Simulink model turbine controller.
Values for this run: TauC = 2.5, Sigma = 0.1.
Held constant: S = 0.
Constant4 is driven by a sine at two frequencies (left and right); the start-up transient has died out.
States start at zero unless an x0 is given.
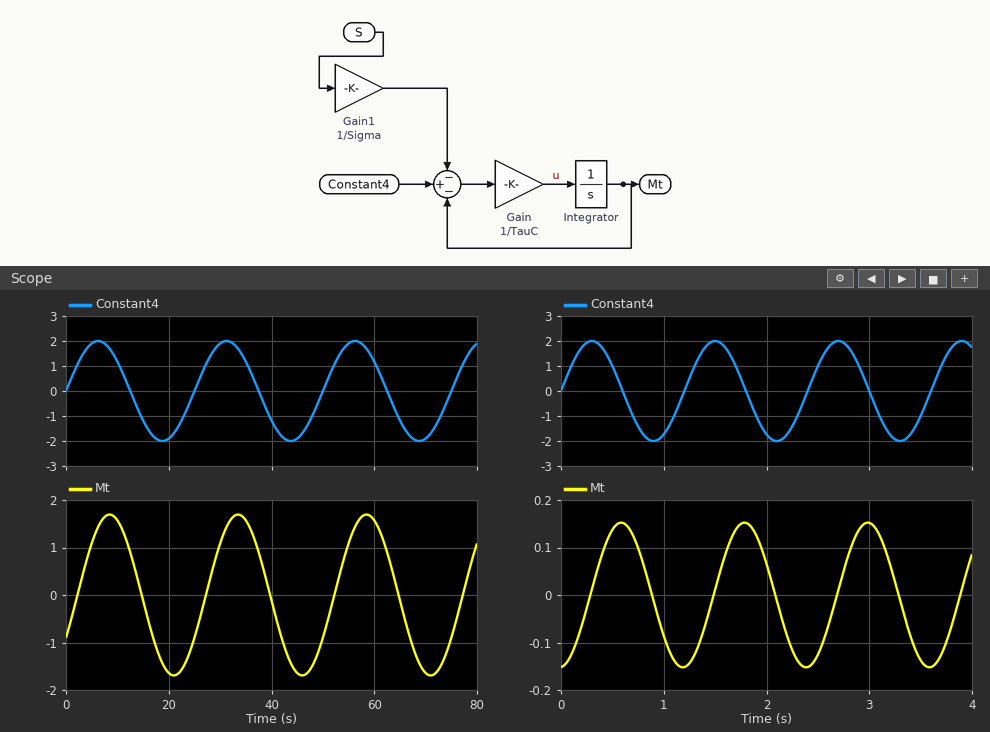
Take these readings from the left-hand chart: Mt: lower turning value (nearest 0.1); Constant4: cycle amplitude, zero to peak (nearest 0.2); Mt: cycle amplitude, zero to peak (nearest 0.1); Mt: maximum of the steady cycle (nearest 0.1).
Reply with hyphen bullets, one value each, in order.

- -1.7
- 2.0
- 1.7
- 1.7
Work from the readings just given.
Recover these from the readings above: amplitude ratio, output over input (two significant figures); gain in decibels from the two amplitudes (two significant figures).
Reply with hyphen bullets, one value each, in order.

- 0.85
- -1.4 dB
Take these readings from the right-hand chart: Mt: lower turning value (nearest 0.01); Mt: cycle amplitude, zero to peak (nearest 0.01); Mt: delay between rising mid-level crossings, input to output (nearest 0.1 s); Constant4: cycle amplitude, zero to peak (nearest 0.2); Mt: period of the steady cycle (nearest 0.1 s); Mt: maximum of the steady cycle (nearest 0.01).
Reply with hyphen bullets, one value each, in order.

- -0.15
- 0.15
- 0.3 s
- 2.0
- 1.2 s
- 0.15
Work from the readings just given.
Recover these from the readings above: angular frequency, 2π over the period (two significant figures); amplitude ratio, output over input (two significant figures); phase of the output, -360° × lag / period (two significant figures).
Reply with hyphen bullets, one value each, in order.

- 5.2 rad/s
- 0.075
- -90°
